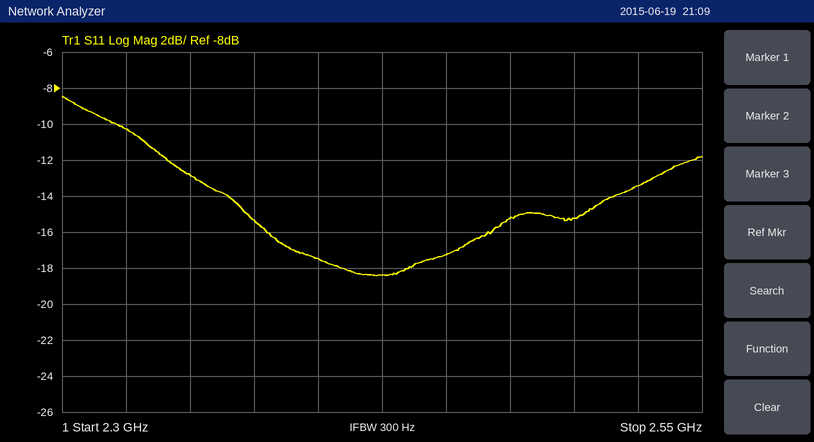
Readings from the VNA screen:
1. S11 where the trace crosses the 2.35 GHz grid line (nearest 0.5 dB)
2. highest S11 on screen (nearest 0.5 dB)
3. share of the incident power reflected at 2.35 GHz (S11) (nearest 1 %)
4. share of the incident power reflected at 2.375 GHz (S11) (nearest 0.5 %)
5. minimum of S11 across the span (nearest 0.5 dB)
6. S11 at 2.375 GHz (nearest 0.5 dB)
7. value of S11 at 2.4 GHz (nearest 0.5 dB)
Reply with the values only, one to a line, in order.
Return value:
-13.0 dB
-8.5 dB
5 %
3.0 %
-18.5 dB
-15.5 dB
-17.5 dB
